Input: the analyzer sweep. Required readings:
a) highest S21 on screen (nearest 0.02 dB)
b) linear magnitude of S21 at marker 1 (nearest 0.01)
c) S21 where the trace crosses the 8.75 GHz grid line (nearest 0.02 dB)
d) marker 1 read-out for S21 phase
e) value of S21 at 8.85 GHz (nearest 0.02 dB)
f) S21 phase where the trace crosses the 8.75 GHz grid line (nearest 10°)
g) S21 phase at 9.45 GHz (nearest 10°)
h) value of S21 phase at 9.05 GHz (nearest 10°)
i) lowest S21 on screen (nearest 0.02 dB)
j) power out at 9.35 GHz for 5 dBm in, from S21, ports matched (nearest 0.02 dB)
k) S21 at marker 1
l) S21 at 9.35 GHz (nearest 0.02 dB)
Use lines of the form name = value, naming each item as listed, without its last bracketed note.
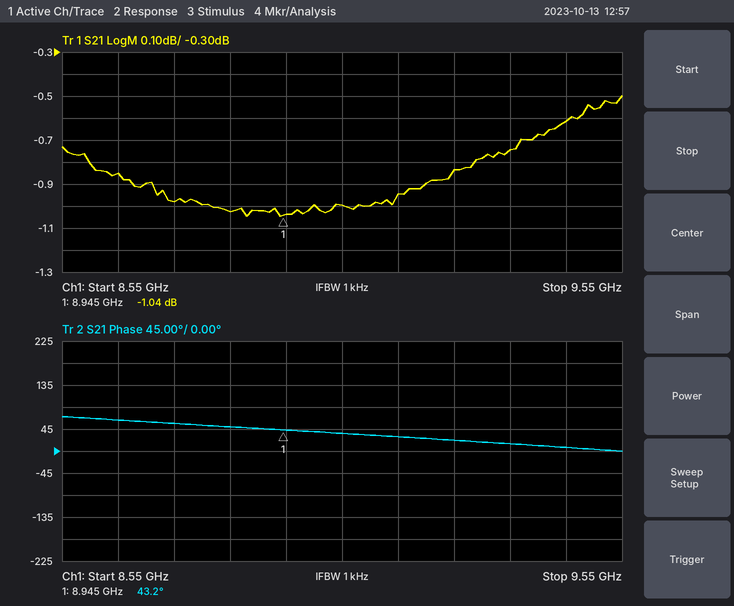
highest S21 on screen = -0.50 dB
linear magnitude of S21 at marker 1 = 0.89
S21 where the trace crosses the 8.75 GHz grid line = -0.98 dB
marker 1 read-out for S21 phase = 43.2°
value of S21 at 8.85 GHz = -1.02 dB
S21 phase where the trace crosses the 8.75 GHz grid line = 60°
S21 phase at 9.45 GHz = 10°
value of S21 phase at 9.05 GHz = 40°
lowest S21 on screen = -1.04 dB
power out at 9.35 GHz for 5 dBm in, from S21, ports matched = 4.26 dBm
S21 at marker 1 = -1.04 dB
S21 at 9.35 GHz = -0.74 dB
